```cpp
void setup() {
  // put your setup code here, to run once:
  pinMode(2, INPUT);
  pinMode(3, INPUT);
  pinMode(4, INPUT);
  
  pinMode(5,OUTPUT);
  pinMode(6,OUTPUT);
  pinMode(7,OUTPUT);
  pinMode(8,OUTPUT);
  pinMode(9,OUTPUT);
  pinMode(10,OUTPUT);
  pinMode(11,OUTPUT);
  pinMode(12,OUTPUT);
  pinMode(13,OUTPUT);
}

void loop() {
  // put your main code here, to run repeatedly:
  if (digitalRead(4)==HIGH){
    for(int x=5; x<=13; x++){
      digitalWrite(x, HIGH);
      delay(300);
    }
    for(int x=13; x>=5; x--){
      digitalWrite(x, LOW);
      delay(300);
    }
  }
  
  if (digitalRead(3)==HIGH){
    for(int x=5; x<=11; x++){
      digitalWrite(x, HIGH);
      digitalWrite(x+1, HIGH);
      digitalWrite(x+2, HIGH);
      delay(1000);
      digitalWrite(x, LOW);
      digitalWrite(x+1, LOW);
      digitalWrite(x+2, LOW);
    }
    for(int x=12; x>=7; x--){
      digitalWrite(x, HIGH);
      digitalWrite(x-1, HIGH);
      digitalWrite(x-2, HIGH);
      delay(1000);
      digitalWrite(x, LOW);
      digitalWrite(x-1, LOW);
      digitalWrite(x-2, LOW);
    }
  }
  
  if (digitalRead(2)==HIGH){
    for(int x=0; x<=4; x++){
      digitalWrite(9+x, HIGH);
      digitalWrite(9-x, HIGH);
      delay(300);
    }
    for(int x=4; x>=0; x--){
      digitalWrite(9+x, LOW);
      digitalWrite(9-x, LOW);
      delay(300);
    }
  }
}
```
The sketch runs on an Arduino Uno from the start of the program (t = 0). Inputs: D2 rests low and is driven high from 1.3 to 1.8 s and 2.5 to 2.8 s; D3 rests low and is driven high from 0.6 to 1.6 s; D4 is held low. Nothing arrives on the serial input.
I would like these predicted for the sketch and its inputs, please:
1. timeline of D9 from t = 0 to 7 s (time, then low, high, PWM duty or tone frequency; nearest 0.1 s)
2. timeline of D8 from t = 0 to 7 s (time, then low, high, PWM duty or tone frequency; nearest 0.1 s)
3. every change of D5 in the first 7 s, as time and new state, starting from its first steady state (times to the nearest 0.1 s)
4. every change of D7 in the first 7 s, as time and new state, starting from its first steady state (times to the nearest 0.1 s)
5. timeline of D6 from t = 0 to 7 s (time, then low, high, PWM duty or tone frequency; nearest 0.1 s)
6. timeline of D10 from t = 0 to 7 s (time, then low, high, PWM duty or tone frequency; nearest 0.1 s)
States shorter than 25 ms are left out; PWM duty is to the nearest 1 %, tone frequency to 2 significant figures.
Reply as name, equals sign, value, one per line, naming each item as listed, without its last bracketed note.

timeline of D9 from t = 0 to 7 s = 0 s low; 2.6 s high; 5.6 s low
timeline of D8 from t = 0 to 7 s = 0 s low; 1.6 s high; 4.6 s low
every change of D5 in the first 7 s, as time and new state, starting from its first steady state = 0 s low; 0.6 s high; 1.6 s low
every change of D7 in the first 7 s, as time and new state, starting from its first steady state = 0 s low; 0.6 s high; 3.6 s low
timeline of D6 from t = 0 to 7 s = 0 s low; 0.6 s high; 2.6 s low
timeline of D10 from t = 0 to 7 s = 0 s low; 3.6 s high; 6.6 s low
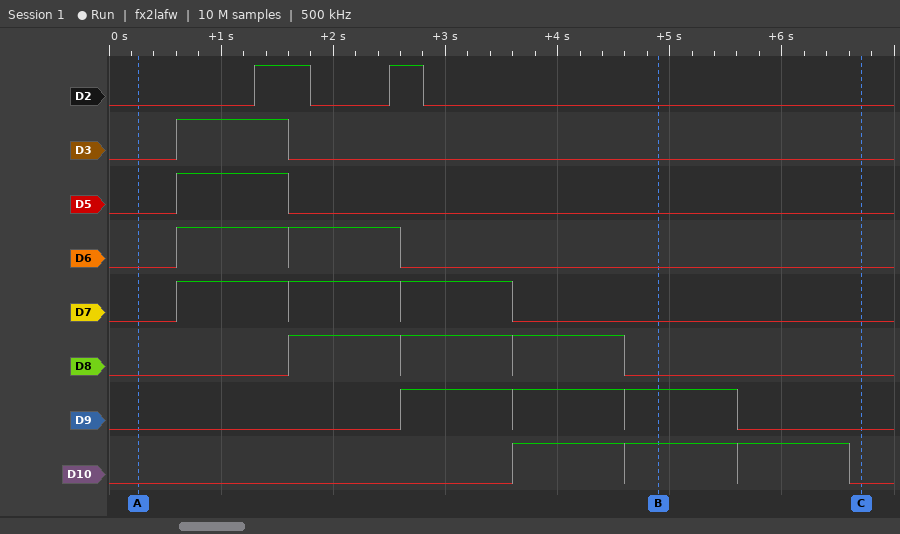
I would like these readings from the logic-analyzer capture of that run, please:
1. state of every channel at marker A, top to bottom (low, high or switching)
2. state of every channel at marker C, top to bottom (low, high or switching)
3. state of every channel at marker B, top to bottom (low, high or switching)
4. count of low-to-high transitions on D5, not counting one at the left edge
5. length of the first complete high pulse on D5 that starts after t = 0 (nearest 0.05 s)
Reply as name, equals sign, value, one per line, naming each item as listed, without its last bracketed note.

state of every channel at marker A, top to bottom = D2 low, D3 low, D5 low, D6 low, D7 low, D8 low, D9 low, D10 low
state of every channel at marker C, top to bottom = D2 low, D3 low, D5 low, D6 low, D7 low, D8 low, D9 low, D10 low
state of every channel at marker B, top to bottom = D2 low, D3 low, D5 low, D6 low, D7 low, D8 low, D9 high, D10 high
count of low-to-high transitions on D5, not counting one at the left edge = 1
length of the first complete high pulse on D5 that starts after t = 0 = 1.00 s
